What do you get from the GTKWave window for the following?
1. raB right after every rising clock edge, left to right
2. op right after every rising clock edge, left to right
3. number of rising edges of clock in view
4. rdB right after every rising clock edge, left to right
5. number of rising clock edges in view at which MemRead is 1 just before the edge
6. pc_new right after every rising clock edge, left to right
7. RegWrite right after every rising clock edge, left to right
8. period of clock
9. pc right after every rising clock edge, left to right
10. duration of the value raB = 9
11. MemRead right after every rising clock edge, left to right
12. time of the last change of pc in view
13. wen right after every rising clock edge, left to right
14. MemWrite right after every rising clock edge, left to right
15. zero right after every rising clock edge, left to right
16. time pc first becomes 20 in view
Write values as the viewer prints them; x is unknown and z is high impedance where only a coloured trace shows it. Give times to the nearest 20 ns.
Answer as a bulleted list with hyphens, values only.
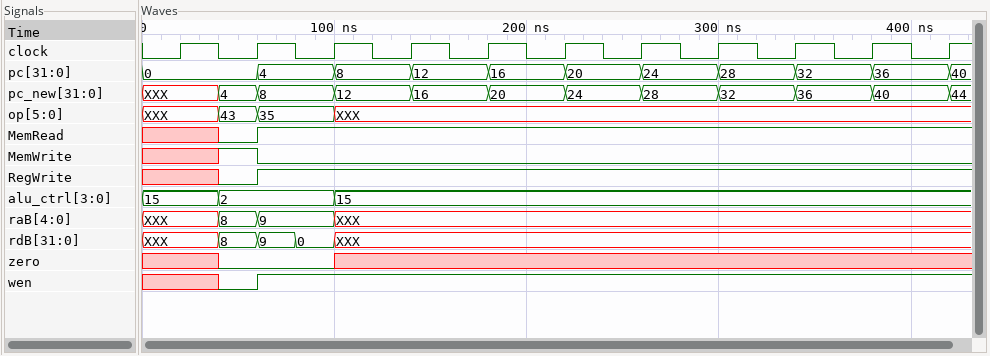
- XXX, 9, XXX, XXX, XXX, XXX, XXX, XXX, XXX, XXX, XXX
- XXX, 35, XXX, XXX, XXX, XXX, XXX, XXX, XXX, XXX, XXX
- 11
- XXX, 9, XXX, XXX, XXX, XXX, XXX, XXX, XXX, XXX, XXX
- 9
- XXX, 8, 12, 16, 20, 24, 28, 32, 36, 40, 44
- x 1 1 1 1 1 1 1 1 1 1
- 40 ns
- 0, 4, 8, 12, 16, 20, 24, 28, 32, 36, 40
- 40 ns
- x 1 1 1 1 1 1 1 1 1 1
- 420 ns
- x 1 1 1 1 1 1 1 1 1 1
- x 0 0 0 0 0 0 0 0 0 0
- x 0 x x x x x x x x x
- 220 ns
